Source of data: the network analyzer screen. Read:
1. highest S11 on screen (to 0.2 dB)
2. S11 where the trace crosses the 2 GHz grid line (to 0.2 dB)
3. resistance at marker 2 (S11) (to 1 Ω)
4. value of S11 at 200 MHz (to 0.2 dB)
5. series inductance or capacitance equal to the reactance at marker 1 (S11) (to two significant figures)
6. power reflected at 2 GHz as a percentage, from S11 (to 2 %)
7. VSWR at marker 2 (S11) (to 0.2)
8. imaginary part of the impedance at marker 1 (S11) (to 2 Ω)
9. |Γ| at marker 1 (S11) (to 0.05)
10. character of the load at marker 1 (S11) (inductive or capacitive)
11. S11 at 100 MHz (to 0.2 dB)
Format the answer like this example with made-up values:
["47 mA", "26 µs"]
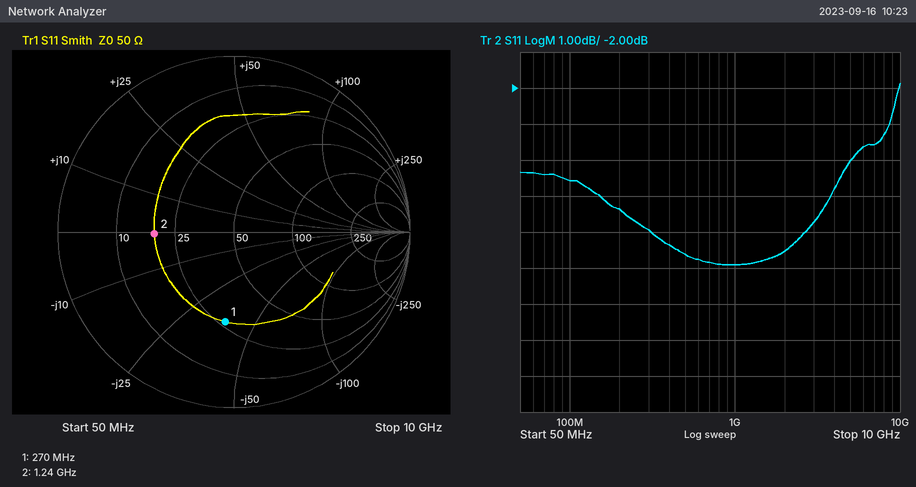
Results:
["-1.8 dB", "-6.6 dB", "19 Ω", "-5.4 dB", "16 pF", "22 %", "2.6", "-38 Ω", "0.50", "capacitive", "-4.6 dB"]
